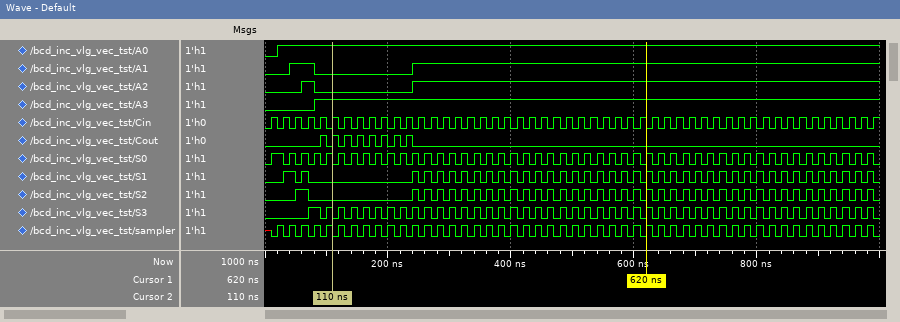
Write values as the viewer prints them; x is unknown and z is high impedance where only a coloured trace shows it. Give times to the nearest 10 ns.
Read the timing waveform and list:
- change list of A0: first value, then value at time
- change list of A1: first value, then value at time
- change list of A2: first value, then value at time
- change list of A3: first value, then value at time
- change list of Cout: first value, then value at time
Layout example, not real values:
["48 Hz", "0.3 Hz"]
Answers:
["0, 1 at 20 ns", "0, 1 at 40 ns, 0 at 80 ns, 1 at 240 ns", "0, 1 at 60 ns, 0 at 80 ns, 1 at 240 ns", "0, 1 at 80 ns", "0, 1 at 90 ns, 0 at 100 ns, 1 at 110 ns, 0 at 120 ns, 1 at 130 ns, 0 at 140 ns, 1 at 150 ns, 0 at 160 ns, 1 at 170 ns, 0 at 180 ns, 1 at 190 ns, 0 at 200 ns, 1 at 210 ns, 0 at 220 ns, 1 at 230 ns, 0 at 240 ns"]
